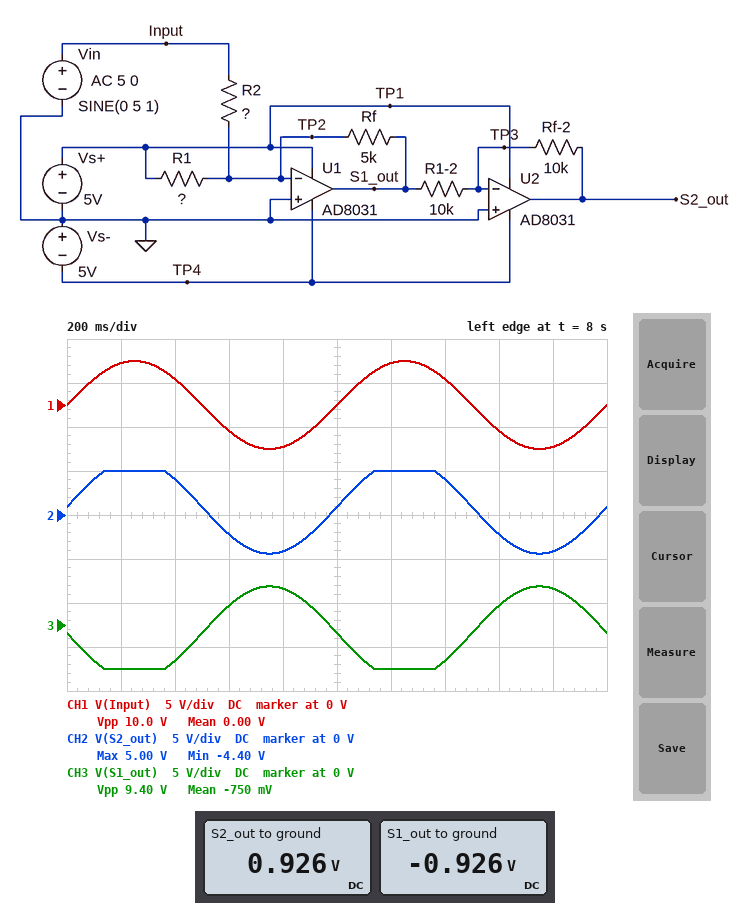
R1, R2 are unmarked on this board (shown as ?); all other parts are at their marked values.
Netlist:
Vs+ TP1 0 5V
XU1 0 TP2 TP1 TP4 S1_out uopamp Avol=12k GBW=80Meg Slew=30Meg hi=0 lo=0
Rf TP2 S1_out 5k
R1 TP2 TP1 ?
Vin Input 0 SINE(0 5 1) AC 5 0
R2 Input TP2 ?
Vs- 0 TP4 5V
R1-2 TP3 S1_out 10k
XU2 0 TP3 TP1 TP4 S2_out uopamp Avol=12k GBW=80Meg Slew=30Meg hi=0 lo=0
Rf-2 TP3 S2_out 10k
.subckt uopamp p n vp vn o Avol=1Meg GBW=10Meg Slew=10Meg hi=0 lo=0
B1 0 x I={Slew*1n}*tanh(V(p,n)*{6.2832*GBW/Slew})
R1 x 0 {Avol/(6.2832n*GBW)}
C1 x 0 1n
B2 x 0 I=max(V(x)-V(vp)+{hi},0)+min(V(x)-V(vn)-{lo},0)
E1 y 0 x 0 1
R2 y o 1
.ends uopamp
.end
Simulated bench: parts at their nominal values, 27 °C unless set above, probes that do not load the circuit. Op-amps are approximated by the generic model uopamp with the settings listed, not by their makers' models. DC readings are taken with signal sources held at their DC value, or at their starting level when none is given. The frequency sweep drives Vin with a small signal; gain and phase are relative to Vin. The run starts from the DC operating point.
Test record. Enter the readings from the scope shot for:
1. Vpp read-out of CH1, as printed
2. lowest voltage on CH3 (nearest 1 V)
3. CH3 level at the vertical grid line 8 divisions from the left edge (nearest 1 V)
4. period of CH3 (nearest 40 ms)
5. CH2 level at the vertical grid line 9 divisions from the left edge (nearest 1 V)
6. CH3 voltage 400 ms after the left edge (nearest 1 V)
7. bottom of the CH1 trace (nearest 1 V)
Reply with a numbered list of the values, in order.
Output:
1. 10.0 V
2. -5 V
3. 2 V
4. 1.00 s
5. -4 V
6. -4 V
7. -5 V
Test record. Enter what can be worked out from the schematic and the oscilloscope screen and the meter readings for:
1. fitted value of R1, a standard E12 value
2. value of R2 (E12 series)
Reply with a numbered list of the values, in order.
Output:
1. 27 kΩ
2. 4.7 kΩ
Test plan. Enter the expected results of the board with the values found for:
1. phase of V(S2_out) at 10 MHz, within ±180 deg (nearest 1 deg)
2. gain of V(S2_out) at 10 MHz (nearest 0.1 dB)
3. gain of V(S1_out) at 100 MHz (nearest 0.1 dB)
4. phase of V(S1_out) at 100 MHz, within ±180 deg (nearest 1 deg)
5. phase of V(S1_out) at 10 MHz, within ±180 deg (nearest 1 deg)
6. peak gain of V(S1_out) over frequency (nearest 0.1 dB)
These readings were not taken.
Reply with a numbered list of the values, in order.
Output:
1. -30 deg
2. -0.1 dB
3. -9.0 dB
4. 110 deg
5. 164 deg
6. 0.5 dB
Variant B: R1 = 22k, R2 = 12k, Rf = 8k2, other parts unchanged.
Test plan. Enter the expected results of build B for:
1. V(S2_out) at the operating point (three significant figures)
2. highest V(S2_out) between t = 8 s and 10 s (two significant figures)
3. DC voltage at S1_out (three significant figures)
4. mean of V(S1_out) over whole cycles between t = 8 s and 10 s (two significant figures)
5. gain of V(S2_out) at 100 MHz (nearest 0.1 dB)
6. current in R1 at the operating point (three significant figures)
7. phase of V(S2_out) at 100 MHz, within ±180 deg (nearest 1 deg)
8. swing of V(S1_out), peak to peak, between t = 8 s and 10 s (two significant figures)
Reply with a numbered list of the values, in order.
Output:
1. 1.86 V
2. 5.0 V
3. -1.86 V
4. -1.8 V
5. -20.7 dB
6. 227 µA
7. -137 deg
8. 6.6 V
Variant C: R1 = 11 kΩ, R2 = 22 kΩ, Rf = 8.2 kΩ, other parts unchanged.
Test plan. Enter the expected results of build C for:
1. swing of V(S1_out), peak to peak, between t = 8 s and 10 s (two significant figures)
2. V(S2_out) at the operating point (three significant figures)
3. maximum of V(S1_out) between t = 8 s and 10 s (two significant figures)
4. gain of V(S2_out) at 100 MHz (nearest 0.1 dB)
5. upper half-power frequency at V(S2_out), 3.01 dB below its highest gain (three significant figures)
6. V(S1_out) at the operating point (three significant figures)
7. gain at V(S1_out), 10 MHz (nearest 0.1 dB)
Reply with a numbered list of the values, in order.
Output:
1. 3.2 V
2. 3.73 V
3. -1.9 V
4. -26.2 dB
5. 25.0 MHz
6. -3.73 V
7. -8.9 dB
